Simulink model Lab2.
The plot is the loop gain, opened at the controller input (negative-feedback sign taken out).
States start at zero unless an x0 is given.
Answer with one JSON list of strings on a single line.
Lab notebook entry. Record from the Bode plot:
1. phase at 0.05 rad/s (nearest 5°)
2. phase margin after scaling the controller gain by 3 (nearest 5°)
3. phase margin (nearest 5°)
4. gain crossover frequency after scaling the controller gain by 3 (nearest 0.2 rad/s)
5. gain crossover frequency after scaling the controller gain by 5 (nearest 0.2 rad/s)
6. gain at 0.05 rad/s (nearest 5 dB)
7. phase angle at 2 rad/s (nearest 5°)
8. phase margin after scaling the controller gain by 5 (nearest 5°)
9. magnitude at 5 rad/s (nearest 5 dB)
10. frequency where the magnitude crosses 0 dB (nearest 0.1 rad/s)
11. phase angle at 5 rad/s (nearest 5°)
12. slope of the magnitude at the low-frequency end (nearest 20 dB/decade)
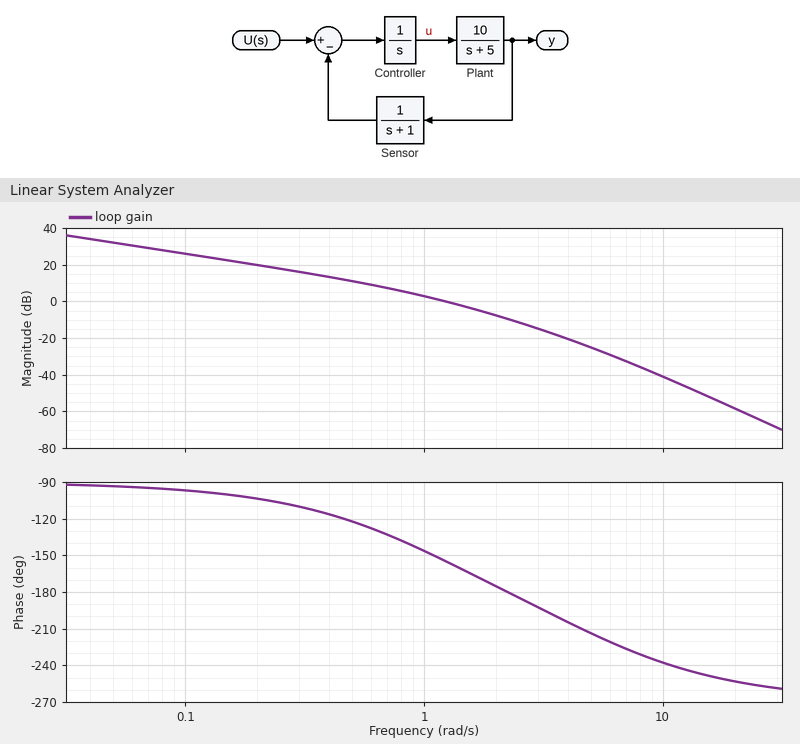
["-95°", "0°", "25°", "2.2 rad/s", "2.8 rad/s", "30 dB", "-175°", "-10°", "-25 dB", "1.2 rad/s", "-215°", "-20 dB/decade"]
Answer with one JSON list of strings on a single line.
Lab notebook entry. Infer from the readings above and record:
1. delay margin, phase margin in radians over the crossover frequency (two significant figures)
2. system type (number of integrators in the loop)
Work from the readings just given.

["0.36 s", "1"]
